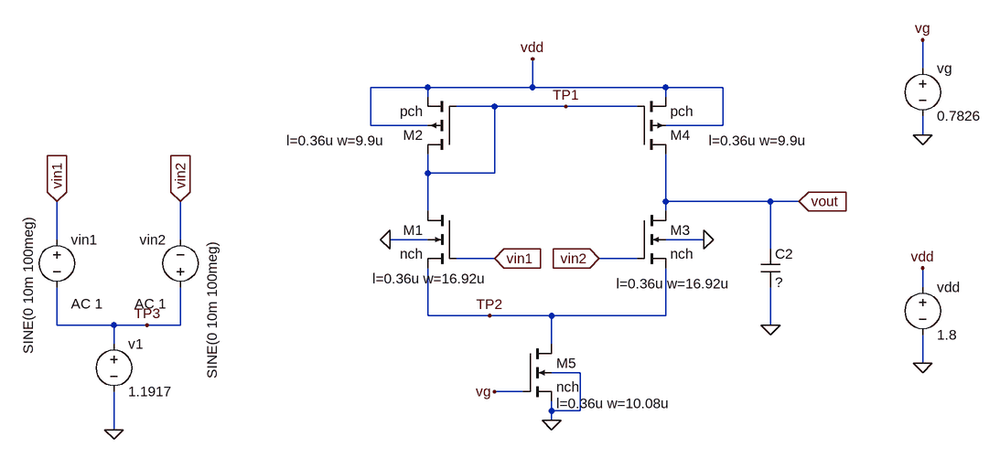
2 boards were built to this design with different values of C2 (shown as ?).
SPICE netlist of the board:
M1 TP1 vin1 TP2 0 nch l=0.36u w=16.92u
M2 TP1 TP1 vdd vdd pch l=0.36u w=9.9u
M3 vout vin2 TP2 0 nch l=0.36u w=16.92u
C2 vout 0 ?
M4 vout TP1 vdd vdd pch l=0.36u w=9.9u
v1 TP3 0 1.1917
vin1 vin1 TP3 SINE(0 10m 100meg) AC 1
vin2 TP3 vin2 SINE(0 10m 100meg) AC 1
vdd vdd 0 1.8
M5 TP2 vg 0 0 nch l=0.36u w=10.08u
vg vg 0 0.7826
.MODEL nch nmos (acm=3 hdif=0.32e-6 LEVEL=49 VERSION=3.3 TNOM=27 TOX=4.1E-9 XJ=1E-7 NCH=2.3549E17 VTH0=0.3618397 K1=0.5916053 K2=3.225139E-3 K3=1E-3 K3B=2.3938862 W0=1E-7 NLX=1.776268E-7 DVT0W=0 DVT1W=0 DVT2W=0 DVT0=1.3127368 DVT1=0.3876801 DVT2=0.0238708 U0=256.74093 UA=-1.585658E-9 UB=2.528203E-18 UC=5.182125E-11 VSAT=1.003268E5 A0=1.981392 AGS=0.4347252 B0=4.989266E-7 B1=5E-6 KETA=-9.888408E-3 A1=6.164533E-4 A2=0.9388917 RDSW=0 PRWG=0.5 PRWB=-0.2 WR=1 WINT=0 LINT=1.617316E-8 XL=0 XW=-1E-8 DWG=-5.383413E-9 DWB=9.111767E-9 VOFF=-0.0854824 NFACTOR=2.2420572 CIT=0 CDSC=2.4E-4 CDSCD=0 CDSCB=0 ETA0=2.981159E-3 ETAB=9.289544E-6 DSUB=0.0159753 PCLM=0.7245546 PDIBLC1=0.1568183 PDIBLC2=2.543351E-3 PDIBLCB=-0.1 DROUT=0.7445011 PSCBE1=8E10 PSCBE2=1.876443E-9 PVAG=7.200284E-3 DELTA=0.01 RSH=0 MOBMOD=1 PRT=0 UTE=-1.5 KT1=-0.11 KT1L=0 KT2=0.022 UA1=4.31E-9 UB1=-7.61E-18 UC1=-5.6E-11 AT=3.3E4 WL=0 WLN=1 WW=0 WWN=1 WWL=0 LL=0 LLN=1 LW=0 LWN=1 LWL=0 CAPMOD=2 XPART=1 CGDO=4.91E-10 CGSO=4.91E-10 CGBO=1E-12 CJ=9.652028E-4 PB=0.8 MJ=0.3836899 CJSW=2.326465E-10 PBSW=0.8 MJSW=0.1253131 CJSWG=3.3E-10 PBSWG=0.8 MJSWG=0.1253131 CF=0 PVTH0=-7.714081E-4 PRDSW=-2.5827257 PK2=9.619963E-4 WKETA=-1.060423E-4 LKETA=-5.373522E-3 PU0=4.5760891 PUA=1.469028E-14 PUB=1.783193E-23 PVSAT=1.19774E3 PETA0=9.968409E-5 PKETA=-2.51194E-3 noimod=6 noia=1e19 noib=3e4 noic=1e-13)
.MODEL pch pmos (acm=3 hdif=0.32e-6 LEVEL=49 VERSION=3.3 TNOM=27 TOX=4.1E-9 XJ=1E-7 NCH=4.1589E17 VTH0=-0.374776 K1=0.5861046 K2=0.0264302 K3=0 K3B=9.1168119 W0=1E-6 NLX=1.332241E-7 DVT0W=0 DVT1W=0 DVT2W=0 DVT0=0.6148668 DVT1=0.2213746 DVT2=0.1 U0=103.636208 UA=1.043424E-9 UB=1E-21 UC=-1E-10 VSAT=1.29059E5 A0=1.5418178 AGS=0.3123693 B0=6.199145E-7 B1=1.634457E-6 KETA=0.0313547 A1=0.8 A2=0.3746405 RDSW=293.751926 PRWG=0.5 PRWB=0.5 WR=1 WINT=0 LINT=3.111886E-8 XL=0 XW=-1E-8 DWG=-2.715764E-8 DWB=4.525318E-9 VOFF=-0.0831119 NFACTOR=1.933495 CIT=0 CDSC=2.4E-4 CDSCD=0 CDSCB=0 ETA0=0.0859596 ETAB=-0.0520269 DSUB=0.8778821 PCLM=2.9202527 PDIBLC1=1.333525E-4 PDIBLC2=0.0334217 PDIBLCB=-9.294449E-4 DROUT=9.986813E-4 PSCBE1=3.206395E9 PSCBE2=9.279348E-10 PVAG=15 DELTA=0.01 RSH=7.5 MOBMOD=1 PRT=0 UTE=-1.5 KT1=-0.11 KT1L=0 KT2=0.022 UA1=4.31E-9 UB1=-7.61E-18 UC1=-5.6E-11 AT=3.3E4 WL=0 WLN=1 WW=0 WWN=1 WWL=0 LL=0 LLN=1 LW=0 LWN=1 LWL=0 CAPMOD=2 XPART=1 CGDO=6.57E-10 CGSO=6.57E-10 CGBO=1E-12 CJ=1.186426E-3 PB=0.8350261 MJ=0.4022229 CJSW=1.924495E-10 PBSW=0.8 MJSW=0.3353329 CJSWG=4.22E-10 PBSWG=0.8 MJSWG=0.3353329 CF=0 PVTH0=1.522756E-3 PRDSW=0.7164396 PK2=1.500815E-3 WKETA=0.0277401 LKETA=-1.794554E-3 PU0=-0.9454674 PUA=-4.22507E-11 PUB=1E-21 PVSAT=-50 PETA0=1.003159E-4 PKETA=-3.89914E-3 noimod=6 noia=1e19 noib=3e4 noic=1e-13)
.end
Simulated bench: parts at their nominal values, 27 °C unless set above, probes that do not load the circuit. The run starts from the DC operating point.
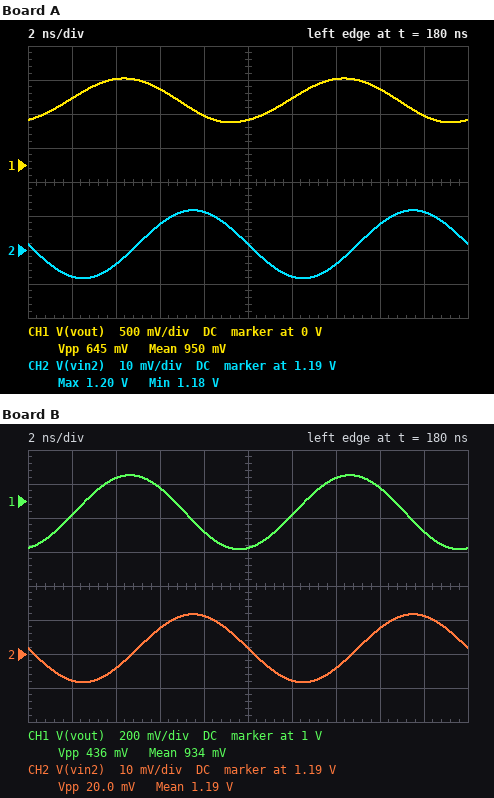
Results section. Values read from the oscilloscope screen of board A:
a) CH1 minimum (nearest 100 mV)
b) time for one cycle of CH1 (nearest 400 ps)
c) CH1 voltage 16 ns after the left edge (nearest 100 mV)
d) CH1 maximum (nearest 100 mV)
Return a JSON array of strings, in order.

["600 mV", "10.0 ns", "1.1 V", "1.3 V"]
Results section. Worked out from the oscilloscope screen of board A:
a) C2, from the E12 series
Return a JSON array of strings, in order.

["120 fF"]
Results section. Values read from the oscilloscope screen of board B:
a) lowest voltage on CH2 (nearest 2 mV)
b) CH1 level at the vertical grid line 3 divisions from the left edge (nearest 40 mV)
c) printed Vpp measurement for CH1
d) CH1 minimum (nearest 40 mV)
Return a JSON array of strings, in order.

["1.182 V", "1.08 V", "436 mV", "720 mV"]
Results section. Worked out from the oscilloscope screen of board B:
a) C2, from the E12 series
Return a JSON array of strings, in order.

["220 fF"]
